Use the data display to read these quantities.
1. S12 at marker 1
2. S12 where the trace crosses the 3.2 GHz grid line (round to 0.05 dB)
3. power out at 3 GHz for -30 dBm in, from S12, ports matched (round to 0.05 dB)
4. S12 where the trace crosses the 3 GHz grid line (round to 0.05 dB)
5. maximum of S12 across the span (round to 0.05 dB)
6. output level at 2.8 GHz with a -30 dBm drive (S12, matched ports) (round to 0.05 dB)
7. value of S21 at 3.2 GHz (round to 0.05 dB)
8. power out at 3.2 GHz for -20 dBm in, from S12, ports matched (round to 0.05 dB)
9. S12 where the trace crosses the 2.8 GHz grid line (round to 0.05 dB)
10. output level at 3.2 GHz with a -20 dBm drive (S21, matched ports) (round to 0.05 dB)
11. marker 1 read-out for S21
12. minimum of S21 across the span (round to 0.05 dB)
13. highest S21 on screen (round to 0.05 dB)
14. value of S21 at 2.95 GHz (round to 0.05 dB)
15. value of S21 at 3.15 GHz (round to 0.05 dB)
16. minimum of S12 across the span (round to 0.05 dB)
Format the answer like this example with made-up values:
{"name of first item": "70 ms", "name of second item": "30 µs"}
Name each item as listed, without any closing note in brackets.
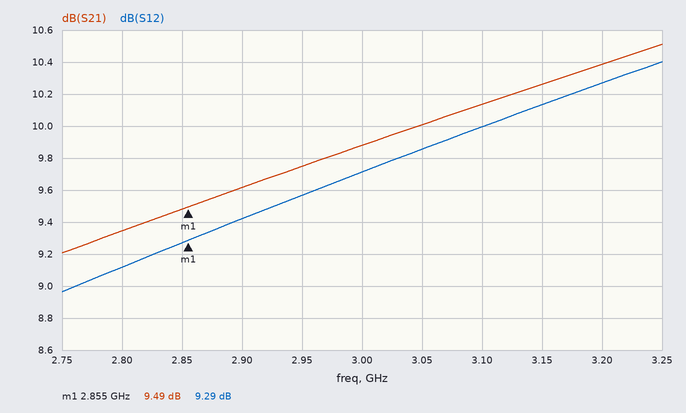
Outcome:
{"S12 at marker 1": "9.29 dB", "S12 where the trace crosses the 3.2 GHz grid line": "10.25 dB", "power out at 3 GHz for -30 dBm in, from S12, ports matched": "-20.30 dBm", "S12 where the trace crosses the 3 GHz grid line": "9.70 dB", "maximum of S12 across the span": "10.40 dB", "output level at 2.8 GHz with a -30 dBm drive (S12, matched ports)": "-20.90 dBm", "value of S21 at 3.2 GHz": "10.40 dB", "power out at 3.2 GHz for -20 dBm in, from S12, ports matched": "-9.75 dBm", "S12 where the trace crosses the 2.8 GHz grid line": "9.10 dB", "output level at 3.2 GHz with a -20 dBm drive (S21, matched ports)": "-9.60 dBm", "marker 1 read-out for S21": "9.49 dB", "minimum of S21 across the span": "9.20 dB", "highest S21 on screen": "10.50 dB", "value of S21 at 2.95 GHz": "9.75 dB", "value of S21 at 3.15 GHz": "10.25 dB", "minimum of S12 across the span": "8.95 dB"}
